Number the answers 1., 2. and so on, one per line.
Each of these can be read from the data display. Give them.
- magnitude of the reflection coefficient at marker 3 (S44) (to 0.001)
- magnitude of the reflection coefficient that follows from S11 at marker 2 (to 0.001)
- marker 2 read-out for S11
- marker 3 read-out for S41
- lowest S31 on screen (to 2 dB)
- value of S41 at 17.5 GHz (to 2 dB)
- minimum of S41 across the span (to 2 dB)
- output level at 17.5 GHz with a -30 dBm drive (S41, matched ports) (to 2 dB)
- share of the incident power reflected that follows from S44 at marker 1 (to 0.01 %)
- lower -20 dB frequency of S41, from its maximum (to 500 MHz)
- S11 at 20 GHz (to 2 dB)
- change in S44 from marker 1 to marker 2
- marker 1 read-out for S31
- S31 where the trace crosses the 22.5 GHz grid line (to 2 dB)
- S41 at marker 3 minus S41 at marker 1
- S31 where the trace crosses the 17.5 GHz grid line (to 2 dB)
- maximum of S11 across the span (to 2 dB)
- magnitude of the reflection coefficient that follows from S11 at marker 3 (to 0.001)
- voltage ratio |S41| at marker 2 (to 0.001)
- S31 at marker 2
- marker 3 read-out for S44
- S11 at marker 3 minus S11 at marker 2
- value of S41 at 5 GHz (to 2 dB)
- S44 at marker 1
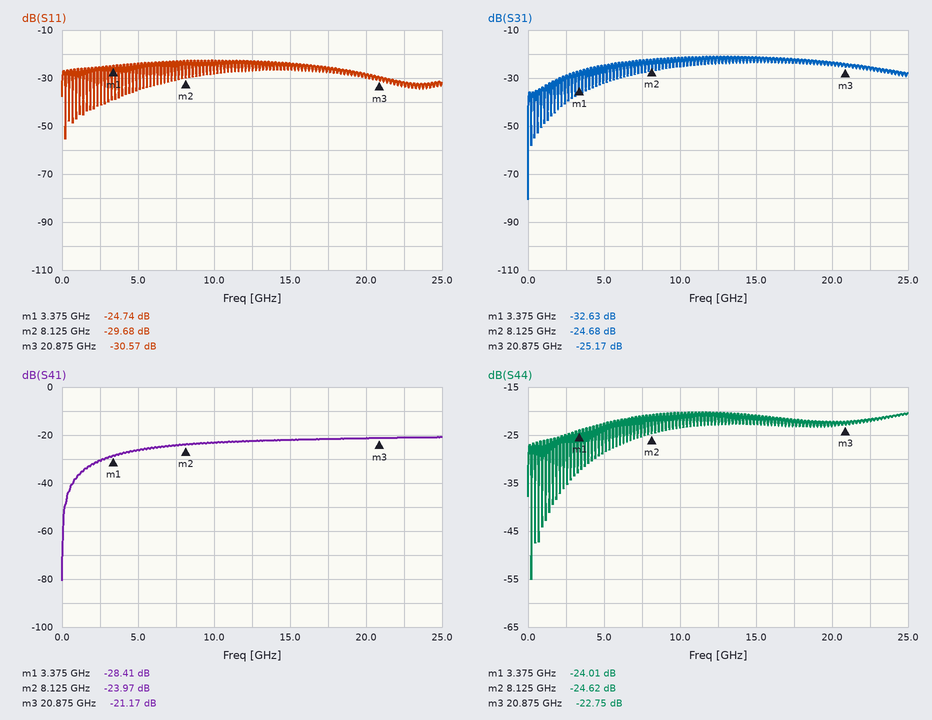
1. 0.073
2. 0.033
3. -29.68 dB
4. -21.17 dB
5. -80 dB
6. -22 dB
7. -80 dB
8. -52 dBm
9. 0.40 %
10. 500 MHz
11. -30 dB
12. -0.61 dB
13. -32.63 dB
14. -26 dB
15. 7.24 dB
16. -22 dB
17. -22 dB
18. 0.030
19. 0.063
20. -24.68 dB
21. -22.75 dB
22. -0.89 dB
23. -26 dB
24. -24.01 dB
